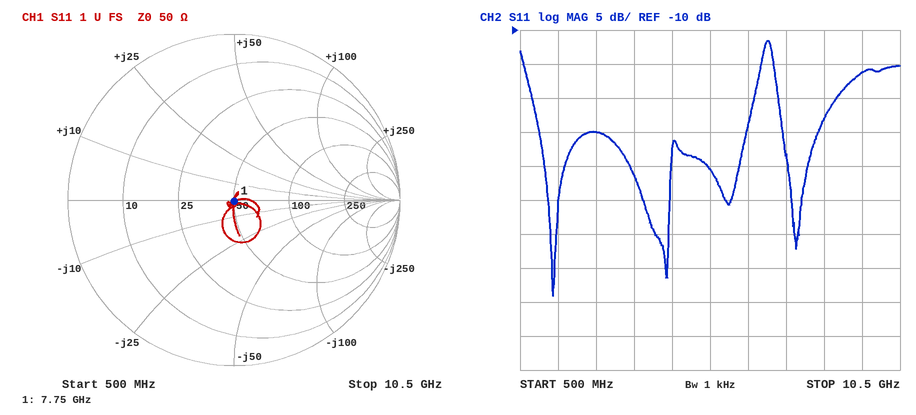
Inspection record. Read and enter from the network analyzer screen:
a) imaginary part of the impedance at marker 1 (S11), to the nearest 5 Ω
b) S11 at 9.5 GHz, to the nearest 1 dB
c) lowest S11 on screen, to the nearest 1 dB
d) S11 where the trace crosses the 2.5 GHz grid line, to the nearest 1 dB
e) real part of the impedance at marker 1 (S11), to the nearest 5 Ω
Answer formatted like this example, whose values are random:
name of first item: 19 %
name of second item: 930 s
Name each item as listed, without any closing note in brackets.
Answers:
imaginary part of the impedance at marker 1 (S11), to the nearest 5 Ω: 0 Ω
S11 at 9.5 GHz, to the nearest 1 dB: -16 dB
lowest S11 on screen, to the nearest 1 dB: -49 dB
S11 where the trace crosses the 2.5 GHz grid line, to the nearest 1 dB: -25 dB
real part of the impedance at marker 1 (S11), to the nearest 5 Ω: 50 Ω
